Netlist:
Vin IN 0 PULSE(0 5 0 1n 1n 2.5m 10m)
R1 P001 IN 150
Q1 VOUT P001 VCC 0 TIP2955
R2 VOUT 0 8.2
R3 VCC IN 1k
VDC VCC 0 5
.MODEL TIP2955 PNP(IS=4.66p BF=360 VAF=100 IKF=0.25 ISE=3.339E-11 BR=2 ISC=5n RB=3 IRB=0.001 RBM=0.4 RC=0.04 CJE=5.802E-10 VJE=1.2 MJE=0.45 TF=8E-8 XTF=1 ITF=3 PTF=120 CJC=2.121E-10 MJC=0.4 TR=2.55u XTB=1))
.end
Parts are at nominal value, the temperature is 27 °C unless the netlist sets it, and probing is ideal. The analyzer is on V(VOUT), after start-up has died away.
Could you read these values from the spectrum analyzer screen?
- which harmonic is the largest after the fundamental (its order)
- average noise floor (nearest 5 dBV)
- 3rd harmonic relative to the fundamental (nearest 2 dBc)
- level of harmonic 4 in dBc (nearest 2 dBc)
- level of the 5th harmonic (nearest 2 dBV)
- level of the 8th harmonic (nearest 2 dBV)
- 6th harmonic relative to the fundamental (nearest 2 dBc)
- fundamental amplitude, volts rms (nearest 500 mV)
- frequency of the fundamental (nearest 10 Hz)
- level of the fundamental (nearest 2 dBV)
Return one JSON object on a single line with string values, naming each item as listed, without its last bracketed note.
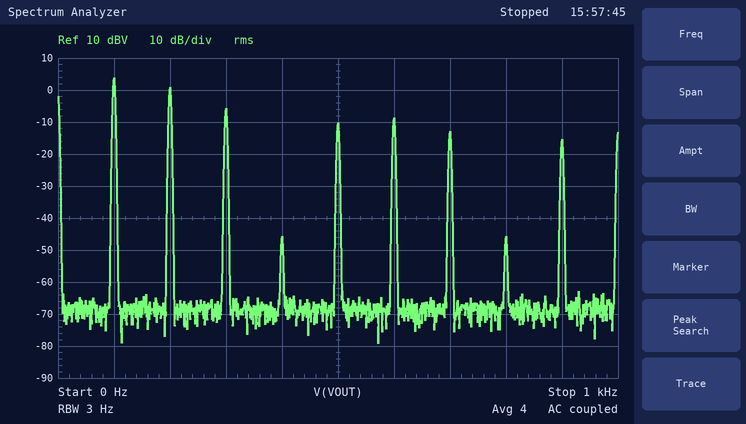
{"which harmonic is the largest after the fundamental": "2", "average noise floor": "-70 dBV", "3rd harmonic relative to the fundamental": "-10 dBc", "level of harmonic 4 in dBc": "-50 dBc", "level of the 5th harmonic": "-10 dBV", "level of the 8th harmonic": "-46 dBV", "6th harmonic relative to the fundamental": "-12 dBc", "fundamental amplitude, volts rms": "1.5 V", "frequency of the fundamental": "100 Hz", "level of the fundamental": "4 dBV"}
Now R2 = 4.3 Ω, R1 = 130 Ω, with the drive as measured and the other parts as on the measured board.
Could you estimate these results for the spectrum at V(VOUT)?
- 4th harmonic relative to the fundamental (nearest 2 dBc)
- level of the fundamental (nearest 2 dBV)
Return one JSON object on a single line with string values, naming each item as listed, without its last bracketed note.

{"4th harmonic relative to the fundamental": "-54 dBc", "level of the fundamental": "4 dBV"}
